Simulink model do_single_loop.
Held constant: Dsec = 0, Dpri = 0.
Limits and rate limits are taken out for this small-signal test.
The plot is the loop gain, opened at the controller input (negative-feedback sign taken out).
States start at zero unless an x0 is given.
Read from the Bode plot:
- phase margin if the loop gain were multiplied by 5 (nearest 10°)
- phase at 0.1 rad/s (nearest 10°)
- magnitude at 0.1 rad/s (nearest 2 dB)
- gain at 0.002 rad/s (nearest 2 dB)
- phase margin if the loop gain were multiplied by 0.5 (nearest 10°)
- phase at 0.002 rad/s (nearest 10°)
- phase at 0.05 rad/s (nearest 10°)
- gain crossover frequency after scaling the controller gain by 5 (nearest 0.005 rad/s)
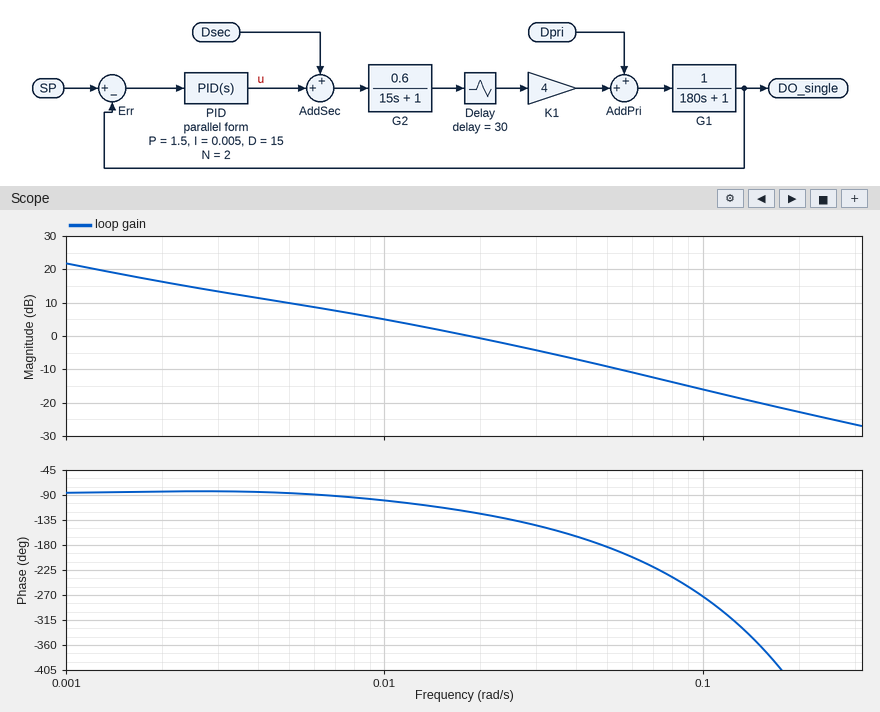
-60°
-270°
-16 dB
16 dB
80°
-80°
-180°
0.080 rad/s
